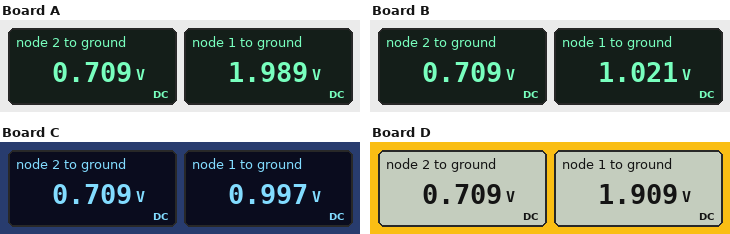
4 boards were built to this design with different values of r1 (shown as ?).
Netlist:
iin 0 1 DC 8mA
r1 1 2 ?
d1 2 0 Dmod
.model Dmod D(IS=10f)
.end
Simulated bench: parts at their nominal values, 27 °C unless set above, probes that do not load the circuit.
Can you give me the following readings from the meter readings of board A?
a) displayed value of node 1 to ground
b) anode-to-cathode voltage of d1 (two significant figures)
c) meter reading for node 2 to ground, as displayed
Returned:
1.989 V
710 mV
0.709 V
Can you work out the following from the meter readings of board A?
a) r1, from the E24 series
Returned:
160 Ω
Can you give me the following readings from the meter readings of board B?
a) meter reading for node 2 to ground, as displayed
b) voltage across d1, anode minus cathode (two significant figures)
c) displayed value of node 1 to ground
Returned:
0.709 V
710 mV
1.021 V
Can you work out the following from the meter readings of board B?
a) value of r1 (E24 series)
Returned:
39 Ω
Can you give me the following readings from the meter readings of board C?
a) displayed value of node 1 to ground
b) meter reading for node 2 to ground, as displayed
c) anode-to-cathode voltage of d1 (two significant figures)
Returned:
0.997 V
0.709 V
710 mV
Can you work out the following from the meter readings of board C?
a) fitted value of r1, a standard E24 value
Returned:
36 Ω
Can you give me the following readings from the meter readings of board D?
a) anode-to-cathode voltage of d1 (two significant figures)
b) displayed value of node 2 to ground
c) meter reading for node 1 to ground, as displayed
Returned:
710 mV
0.709 V
1.909 V
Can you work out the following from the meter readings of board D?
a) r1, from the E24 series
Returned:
150 Ω
